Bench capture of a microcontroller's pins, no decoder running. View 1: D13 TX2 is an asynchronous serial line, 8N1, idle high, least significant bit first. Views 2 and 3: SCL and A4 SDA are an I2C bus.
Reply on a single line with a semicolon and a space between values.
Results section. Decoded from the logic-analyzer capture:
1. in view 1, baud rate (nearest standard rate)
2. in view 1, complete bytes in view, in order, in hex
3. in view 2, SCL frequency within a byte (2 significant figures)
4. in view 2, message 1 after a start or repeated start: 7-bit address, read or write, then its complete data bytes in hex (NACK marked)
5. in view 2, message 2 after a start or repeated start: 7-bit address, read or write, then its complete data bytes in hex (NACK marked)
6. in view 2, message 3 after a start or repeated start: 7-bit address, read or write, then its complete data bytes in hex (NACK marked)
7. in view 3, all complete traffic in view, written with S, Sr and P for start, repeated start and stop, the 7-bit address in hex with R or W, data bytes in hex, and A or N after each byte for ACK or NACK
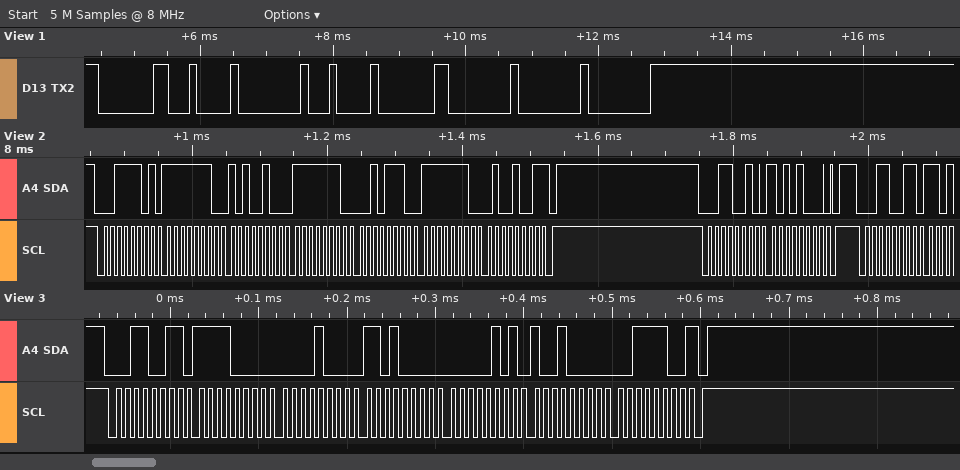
9600 baud; 80 04 00 04 80 00 00 00; 100 kHz; 0x1E read: FE A4 FE 2E FE 49 NACK; 0x19 write: A8; 0x19 read; S 19R A F0 A 08 A D0 A 05 A 90 A 3C N P
